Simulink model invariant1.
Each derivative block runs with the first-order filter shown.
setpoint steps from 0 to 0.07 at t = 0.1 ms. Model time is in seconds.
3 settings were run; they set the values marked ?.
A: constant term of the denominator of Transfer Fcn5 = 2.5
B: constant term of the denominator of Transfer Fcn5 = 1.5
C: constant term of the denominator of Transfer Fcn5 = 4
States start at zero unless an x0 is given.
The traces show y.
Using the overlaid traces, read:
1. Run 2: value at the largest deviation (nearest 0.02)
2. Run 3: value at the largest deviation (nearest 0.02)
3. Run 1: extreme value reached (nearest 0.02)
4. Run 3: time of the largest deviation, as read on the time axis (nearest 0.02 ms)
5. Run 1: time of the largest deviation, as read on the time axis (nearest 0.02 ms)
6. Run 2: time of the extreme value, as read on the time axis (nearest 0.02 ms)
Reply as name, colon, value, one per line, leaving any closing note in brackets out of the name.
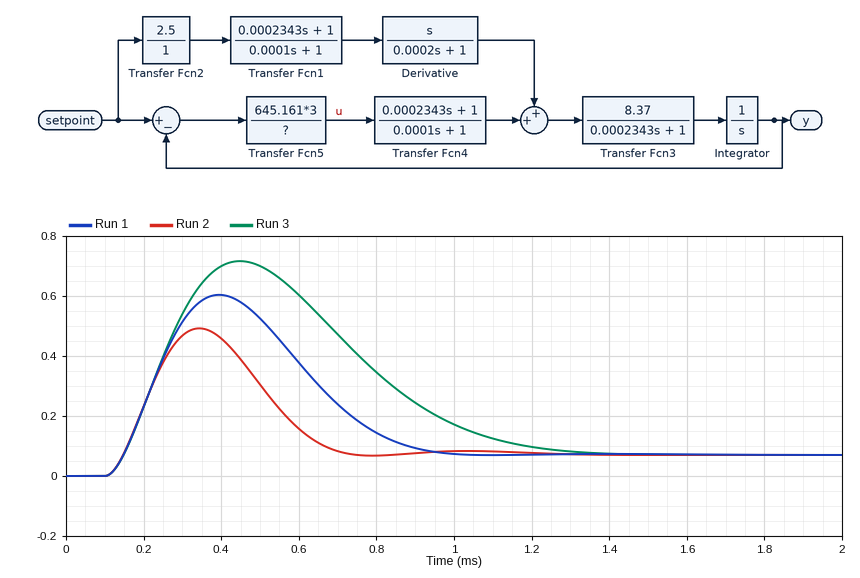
Run 2: value at the largest deviation: 0.50
Run 3: value at the largest deviation: 0.72
Run 1: extreme value reached: 0.60
Run 3: time of the largest deviation, as read on the time axis: 0.44 ms
Run 1: time of the largest deviation, as read on the time axis: 0.40 ms
Run 2: time of the extreme value, as read on the time axis: 0.34 ms
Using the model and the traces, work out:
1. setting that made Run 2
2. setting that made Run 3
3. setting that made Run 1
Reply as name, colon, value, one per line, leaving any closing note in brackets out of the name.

setting that made Run 2: B
setting that made Run 3: C
setting that made Run 1: A
